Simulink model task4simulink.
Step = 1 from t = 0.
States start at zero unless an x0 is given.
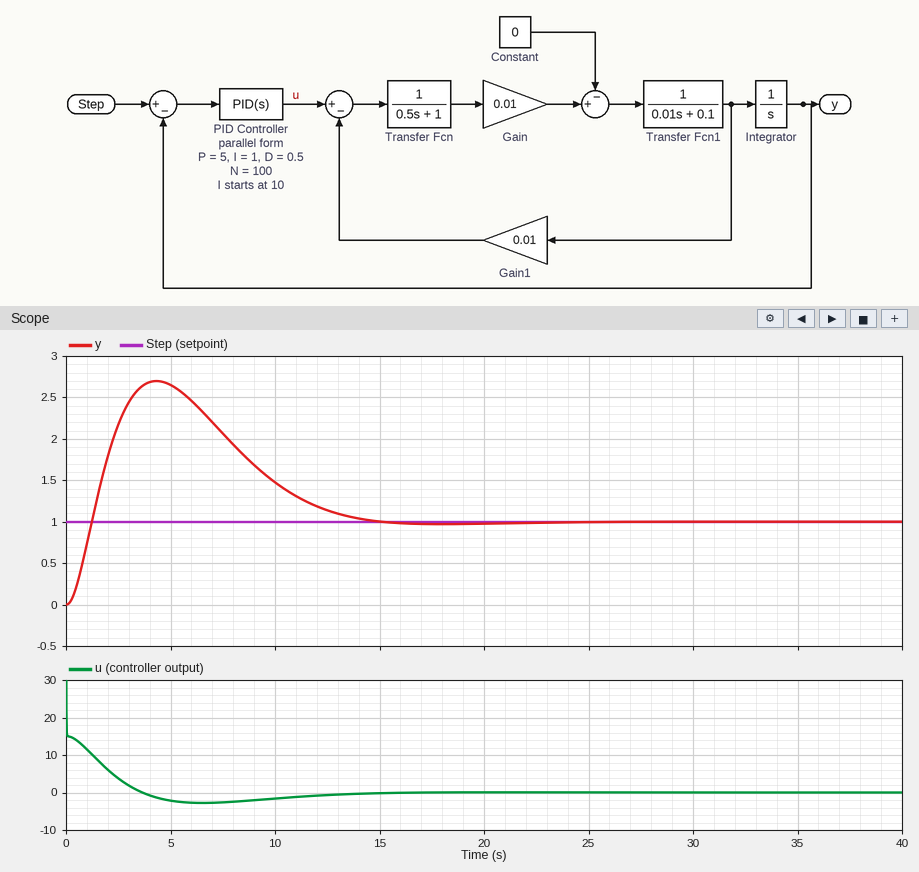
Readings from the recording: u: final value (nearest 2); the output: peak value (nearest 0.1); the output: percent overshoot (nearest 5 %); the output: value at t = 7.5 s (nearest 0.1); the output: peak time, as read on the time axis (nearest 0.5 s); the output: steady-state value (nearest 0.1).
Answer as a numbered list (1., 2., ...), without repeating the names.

1. 0
2. 2.7
3. 170 %
4. 2.1
5. 4.5 s
6. 1.0
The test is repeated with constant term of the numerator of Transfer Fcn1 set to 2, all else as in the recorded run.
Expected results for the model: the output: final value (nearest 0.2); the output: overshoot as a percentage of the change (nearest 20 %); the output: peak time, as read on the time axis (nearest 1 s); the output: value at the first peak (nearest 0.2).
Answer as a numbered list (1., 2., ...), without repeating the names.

1. 1.0
2. 200 %
3. 3 s
4. 3.0
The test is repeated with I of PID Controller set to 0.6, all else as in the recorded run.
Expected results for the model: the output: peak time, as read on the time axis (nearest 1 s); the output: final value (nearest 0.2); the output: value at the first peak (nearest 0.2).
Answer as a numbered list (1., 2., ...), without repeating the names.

1. 5 s
2. 1.0
3. 2.8
